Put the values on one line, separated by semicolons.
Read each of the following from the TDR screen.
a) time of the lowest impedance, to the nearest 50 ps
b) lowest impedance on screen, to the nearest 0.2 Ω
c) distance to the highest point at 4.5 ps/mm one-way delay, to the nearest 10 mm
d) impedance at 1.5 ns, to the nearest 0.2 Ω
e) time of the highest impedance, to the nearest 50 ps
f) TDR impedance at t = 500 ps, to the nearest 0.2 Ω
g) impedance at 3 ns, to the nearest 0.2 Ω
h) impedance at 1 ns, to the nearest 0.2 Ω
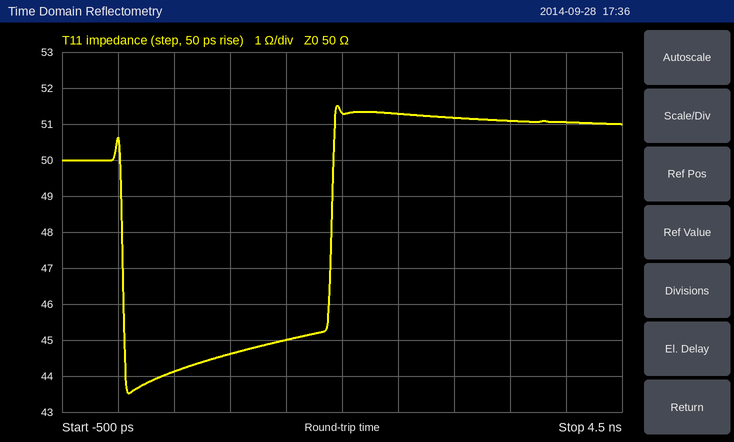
100 ps; 43.6 Ω; 220 mm; 45.0 Ω; 1.95 ns; 44.2 Ω; 51.2 Ω; 44.6 Ω
